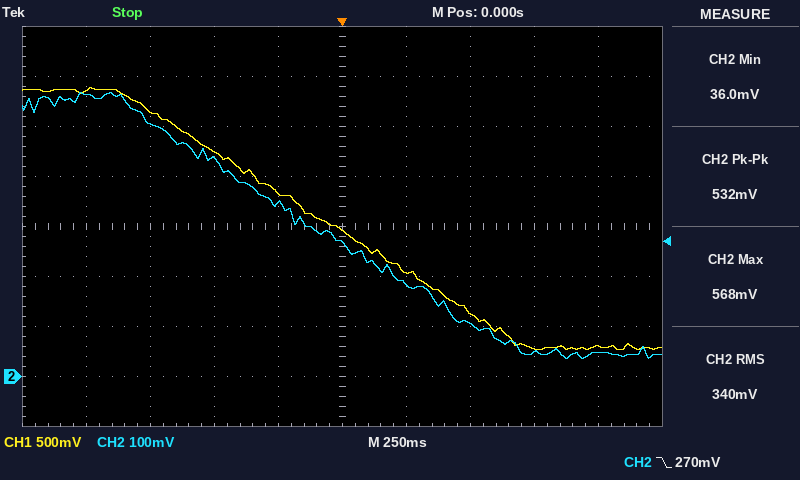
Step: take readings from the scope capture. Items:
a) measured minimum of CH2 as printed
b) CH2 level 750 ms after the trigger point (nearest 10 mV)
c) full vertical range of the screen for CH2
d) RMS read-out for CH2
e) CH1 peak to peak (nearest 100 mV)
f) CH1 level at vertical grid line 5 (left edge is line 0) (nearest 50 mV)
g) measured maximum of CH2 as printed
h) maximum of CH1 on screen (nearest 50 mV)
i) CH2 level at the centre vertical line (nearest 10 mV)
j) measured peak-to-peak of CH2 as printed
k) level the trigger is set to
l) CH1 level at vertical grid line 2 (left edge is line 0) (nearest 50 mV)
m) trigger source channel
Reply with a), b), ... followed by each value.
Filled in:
a) 36.0 mV
b) 50 mV
c) 800 mV
d) 340 mV
e) 2.60 V
f) 1.45 V
g) 568 mV
h) 2.90 V
i) 270 mV
j) 532 mV
k) 270 mV
l) 2.65 V
m) CH2
